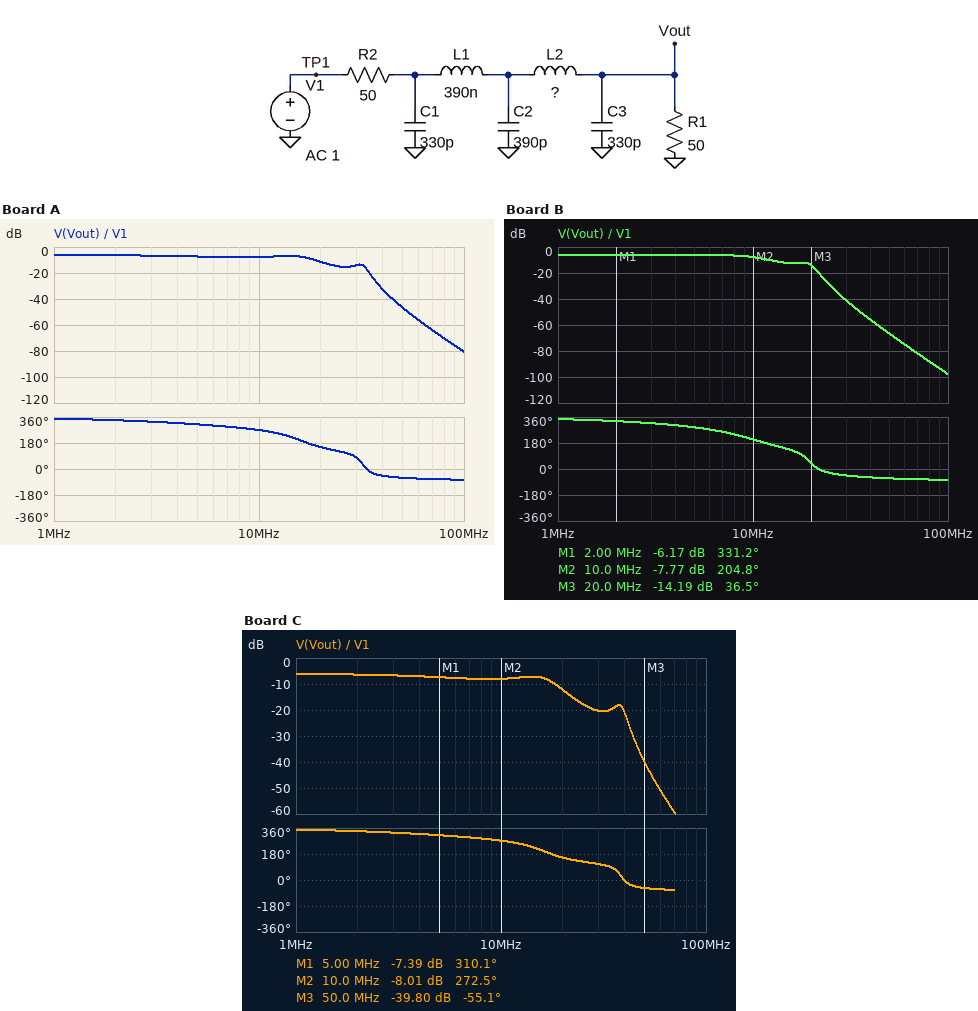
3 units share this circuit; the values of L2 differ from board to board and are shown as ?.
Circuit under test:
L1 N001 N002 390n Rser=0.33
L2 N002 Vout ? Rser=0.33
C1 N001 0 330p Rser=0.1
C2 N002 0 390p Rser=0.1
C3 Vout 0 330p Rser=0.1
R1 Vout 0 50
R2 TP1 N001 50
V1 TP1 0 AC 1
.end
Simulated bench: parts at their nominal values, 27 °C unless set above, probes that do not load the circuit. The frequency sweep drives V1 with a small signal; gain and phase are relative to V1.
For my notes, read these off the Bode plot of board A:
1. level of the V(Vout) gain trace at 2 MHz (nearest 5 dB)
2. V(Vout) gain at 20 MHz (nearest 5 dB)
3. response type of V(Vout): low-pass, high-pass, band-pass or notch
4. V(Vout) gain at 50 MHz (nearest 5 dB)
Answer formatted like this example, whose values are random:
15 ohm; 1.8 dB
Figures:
-5 dB; -10 dB; low-pass; -45 dB
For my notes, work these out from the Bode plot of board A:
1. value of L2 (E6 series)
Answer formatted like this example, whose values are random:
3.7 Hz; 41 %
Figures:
150 nH
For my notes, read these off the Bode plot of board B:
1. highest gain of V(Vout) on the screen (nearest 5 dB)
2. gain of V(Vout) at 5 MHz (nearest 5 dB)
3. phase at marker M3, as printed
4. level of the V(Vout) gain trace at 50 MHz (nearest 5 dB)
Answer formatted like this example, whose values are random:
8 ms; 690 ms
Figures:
-5 dB; -5 dB; 36.5 deg; -65 dB
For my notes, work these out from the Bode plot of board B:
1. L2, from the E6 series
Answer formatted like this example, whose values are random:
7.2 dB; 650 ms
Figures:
1 µH
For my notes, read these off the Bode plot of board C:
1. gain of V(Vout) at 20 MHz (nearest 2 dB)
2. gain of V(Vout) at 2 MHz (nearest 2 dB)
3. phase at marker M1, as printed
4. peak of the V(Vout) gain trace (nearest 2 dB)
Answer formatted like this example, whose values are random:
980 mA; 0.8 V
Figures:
-12 dB; -6 dB; 310.1 deg; -6 dB
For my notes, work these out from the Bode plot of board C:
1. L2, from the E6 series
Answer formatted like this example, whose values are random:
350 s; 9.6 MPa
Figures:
100 nH
